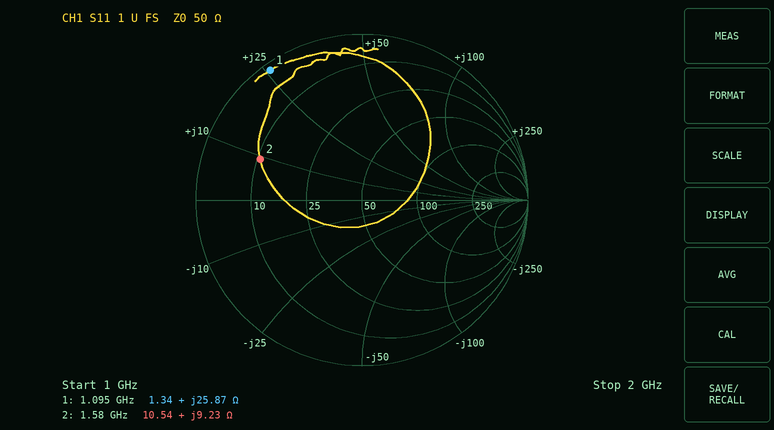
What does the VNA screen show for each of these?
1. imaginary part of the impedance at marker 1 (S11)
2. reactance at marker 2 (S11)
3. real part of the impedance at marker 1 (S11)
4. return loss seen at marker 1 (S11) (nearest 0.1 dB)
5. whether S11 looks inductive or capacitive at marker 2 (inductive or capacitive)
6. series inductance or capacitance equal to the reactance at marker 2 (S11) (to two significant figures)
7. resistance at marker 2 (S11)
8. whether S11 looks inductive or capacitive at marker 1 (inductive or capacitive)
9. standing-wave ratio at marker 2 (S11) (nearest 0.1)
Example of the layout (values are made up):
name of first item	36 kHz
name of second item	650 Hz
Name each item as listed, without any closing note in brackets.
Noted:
imaginary part of the impedance at marker 1	+25.87 Ω
reactance at marker 2	+9.23 Ω
real part of the impedance at marker 1	1.34 Ω
return loss seen at marker 1 (S11)	0.4 dB
whether S11 looks inductive or capacitive at marker 2	inductive
series inductance or capacitance equal to the reactance at marker 2 (S11)	930 pH
resistance at marker 2	10.54 Ω
whether S11 looks inductive or capacitive at marker 1	inductive
standing-wave ratio at marker 2 (S11)	4.9
